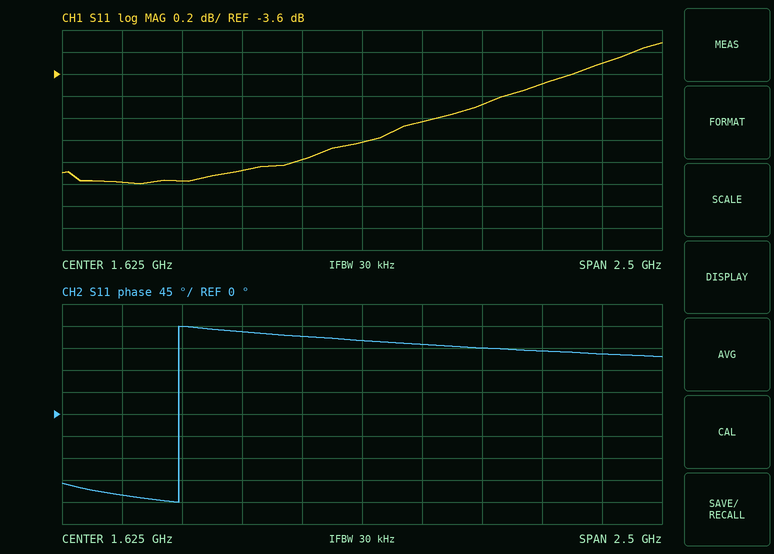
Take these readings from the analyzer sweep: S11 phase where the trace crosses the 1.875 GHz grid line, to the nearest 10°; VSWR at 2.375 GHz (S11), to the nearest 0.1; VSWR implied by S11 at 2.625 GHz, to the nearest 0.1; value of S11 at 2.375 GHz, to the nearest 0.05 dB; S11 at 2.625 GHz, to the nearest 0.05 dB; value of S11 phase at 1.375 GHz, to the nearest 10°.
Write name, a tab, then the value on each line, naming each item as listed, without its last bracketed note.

S11 phase where the trace crosses the 1.875 GHz grid line, to the nearest 10°	140°
VSWR at 2.375 GHz (S11), to the nearest 0.1	4.8
VSWR implied by S11 at 2.625 GHz, to the nearest 0.1	5.0
value of S11 at 2.375 GHz, to the nearest 0.05 dB	-3.70 dB
S11 at 2.625 GHz, to the nearest 0.05 dB	-3.50 dB
value of S11 phase at 1.375 GHz, to the nearest 10°	160°
